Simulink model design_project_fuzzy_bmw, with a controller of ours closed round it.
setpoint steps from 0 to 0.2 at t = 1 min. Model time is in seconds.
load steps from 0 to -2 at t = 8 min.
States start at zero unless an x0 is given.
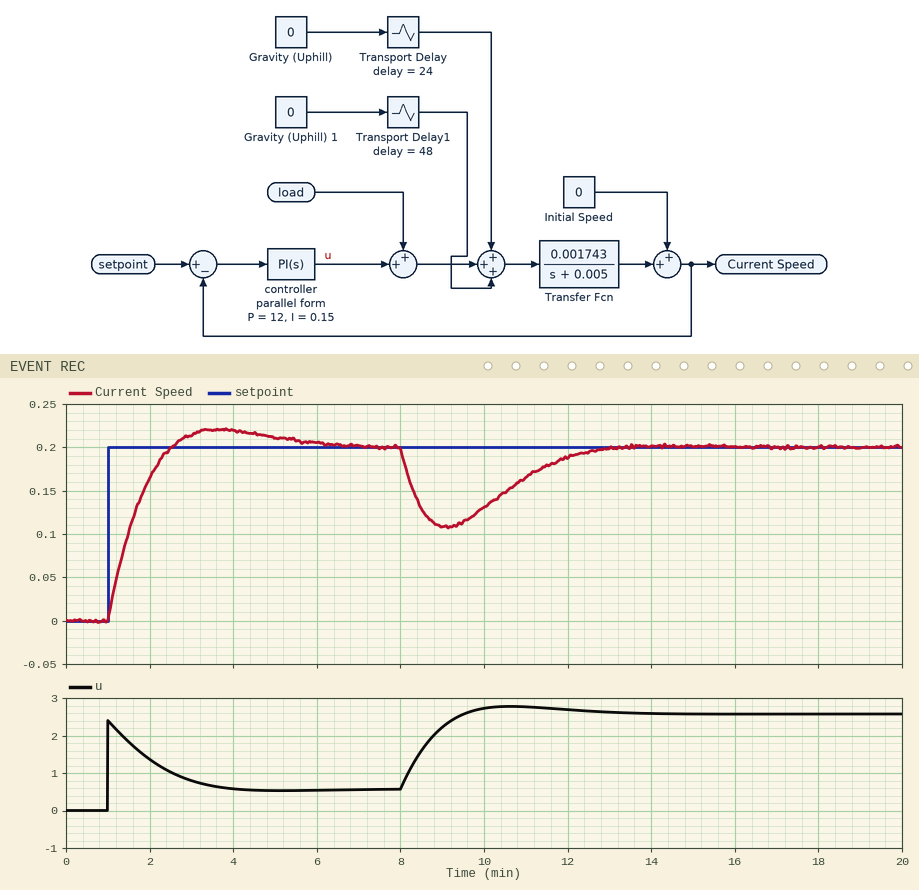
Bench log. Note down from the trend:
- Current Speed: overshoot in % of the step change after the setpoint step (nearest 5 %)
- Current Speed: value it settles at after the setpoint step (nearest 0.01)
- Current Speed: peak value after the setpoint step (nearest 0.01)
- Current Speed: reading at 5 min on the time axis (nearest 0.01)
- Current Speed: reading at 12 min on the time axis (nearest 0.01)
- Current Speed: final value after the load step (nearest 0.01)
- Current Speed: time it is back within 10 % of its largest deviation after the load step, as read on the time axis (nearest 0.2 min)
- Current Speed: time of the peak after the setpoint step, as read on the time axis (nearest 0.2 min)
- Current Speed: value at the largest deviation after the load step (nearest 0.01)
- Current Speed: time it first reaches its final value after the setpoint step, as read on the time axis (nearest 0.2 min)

10 %
0.20
0.22
0.21
0.19
0.20
12.2 min
3.6 min
0.11
2.6 min
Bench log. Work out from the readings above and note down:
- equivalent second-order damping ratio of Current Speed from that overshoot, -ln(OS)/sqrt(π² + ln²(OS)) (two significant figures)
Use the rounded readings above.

0.59
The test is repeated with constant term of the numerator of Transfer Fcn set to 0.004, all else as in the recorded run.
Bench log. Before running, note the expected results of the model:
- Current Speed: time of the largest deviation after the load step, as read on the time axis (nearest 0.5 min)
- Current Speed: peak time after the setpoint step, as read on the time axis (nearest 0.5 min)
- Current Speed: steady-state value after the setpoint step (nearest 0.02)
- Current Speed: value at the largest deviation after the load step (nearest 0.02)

8.5 min
2.5 min
0.20
0.08
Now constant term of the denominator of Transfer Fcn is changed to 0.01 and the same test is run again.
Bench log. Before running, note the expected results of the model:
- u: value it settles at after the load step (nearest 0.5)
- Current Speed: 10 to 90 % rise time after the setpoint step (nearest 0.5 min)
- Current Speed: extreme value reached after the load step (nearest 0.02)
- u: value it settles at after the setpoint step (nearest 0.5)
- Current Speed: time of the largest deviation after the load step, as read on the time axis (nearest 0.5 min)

3.0
1.5 min
0.12
1.0
9.0 min
